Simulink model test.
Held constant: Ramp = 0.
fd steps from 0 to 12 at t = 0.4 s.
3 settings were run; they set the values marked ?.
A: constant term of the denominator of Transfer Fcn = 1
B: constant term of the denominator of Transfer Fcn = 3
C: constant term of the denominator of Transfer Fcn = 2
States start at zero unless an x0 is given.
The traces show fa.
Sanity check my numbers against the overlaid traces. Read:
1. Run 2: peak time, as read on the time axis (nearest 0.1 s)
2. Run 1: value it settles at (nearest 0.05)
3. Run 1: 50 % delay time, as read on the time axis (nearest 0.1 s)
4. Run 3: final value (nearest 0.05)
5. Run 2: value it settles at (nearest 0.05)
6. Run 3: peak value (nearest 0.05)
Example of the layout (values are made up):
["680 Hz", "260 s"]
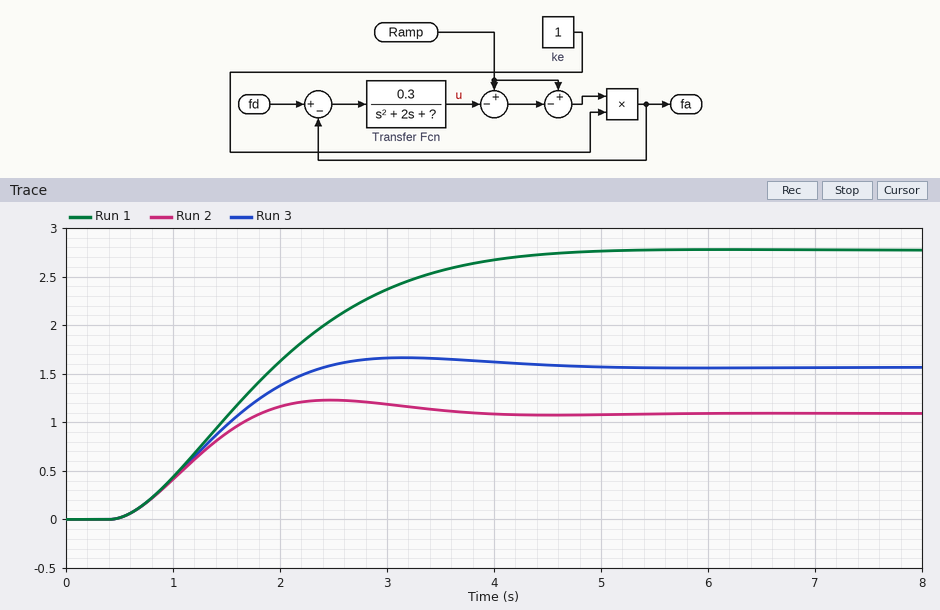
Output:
["2.5 s", "2.75", "1.8 s", "1.55", "1.10", "1.65"]
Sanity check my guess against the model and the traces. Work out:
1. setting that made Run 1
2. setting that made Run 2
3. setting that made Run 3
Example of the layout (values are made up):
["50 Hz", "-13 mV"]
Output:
["A", "B", "C"]
